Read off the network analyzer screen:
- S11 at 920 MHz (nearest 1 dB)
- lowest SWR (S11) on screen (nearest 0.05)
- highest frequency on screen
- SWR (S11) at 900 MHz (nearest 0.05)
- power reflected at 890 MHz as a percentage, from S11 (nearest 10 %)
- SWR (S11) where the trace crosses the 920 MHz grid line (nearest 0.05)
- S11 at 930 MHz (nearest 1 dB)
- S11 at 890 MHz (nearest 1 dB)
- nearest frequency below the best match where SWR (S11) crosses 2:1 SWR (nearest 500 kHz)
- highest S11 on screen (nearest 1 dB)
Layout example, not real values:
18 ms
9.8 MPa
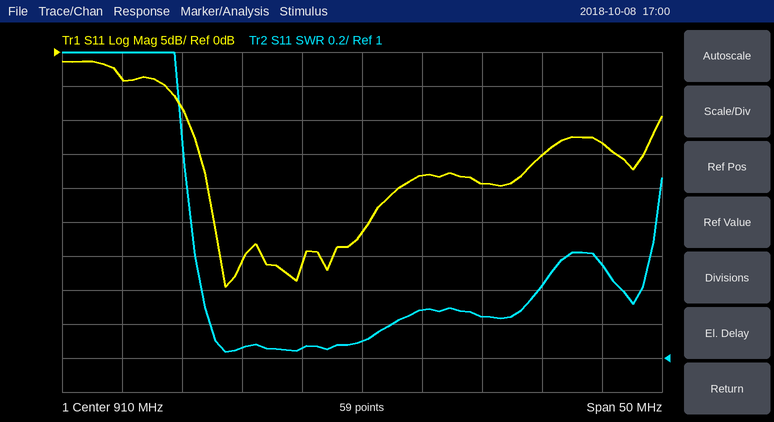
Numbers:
-19 dB
1.05
935 MHz
1.05
40 %
1.25
-13 dB
-4 dB
895.5 MHz
-1 dB
